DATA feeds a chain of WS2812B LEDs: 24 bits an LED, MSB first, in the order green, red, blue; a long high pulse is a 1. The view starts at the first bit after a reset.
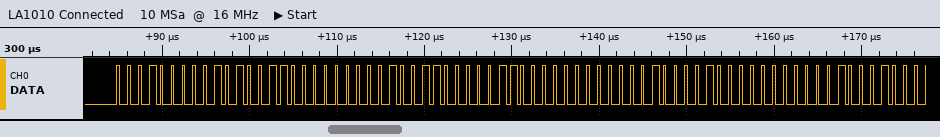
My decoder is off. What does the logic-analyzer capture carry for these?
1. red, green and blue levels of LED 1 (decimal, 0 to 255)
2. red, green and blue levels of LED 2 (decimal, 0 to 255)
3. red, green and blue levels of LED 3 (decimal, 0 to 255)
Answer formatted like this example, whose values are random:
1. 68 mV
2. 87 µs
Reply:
1. 83, 16, 0
2. 24, 76, 0
3. 0, 66, 34
